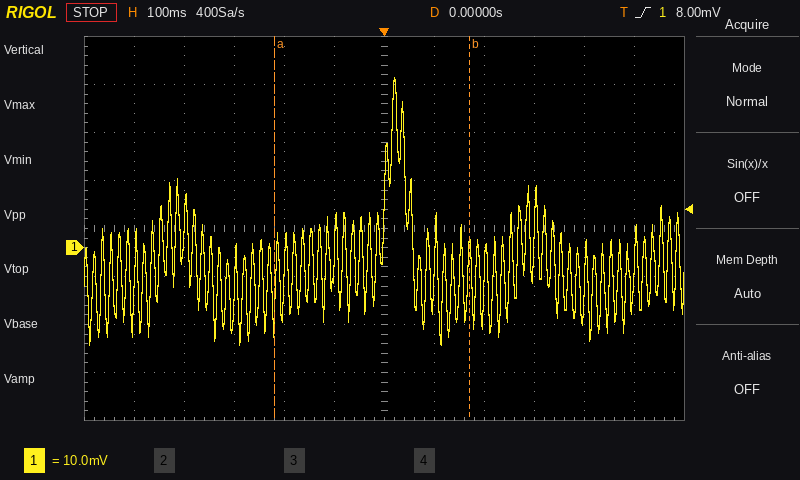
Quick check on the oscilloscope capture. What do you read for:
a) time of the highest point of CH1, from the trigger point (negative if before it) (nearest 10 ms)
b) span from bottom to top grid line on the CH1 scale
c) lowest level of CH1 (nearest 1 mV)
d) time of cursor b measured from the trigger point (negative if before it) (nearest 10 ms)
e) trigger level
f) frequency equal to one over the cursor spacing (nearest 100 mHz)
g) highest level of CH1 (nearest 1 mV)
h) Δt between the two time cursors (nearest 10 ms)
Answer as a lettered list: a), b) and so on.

a) +20 ms
b) 80 mV
c) -20 mV
d) +170 ms
e) 8.00 mV
f) 2.6 Hz
g) 35 mV
h) 390 ms
